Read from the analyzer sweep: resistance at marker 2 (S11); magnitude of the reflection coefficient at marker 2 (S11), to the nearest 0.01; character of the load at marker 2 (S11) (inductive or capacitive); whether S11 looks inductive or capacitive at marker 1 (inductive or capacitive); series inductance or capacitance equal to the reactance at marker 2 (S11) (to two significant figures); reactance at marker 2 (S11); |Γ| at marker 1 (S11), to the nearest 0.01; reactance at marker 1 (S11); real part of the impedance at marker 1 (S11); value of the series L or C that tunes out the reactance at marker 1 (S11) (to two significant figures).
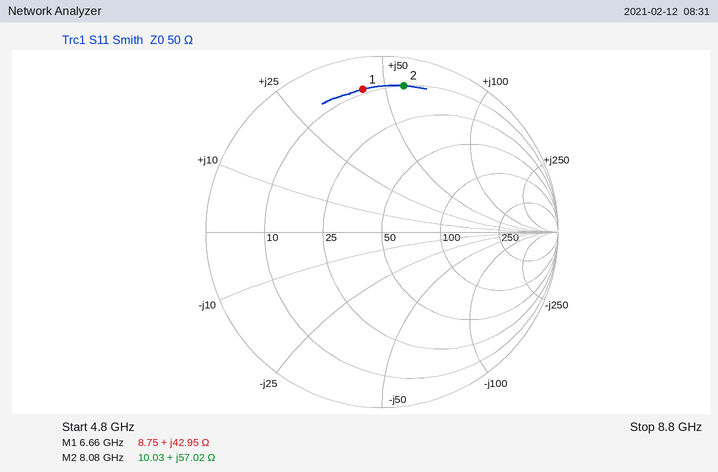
10.03 Ω
0.84
inductive
inductive
1.1 nH
+57.02 Ω
0.82
+42.95 Ω
8.75 Ω
560 fF
